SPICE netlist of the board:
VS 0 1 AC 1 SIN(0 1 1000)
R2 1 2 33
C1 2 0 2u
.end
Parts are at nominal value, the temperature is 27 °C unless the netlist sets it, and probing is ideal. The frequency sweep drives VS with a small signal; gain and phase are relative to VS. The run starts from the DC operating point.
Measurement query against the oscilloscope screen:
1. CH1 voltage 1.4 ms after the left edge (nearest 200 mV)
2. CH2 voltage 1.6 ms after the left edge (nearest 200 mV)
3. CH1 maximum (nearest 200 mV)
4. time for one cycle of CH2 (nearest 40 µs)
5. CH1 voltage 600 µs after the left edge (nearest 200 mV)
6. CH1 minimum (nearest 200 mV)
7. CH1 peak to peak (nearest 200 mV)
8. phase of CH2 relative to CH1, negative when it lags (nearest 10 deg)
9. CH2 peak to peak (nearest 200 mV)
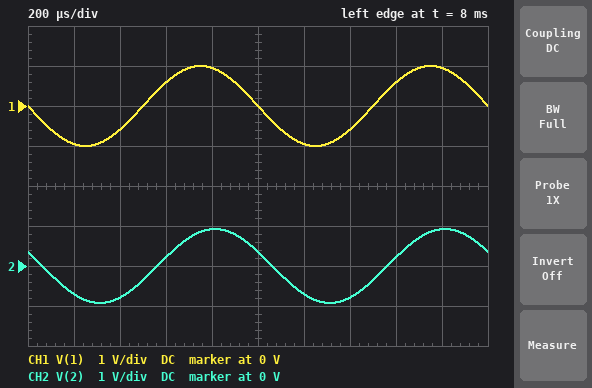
-600 mV
200 mV
1.0 V
1.00 ms
600 mV
-1.0 V
2.0 V
-20 deg
1.8 V
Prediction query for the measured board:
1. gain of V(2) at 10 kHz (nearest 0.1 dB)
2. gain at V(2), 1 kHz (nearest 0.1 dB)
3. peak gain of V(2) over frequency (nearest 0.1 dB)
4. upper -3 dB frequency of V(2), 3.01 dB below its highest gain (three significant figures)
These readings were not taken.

-12.6 dB
-0.7 dB
0 dB
2.41 kHz
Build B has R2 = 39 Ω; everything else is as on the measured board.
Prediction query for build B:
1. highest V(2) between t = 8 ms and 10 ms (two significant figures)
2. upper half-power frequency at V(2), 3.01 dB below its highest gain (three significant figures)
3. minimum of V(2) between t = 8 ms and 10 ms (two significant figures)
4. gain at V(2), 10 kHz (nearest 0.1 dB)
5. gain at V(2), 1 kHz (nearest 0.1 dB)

900 mV
2.04 kHz
-900 mV
-14.0 dB
-0.9 dB
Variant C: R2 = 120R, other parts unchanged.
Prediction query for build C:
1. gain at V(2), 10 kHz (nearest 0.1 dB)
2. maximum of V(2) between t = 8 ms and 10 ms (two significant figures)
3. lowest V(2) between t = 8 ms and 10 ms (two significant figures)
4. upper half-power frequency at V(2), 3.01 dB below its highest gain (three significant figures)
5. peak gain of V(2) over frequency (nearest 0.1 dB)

-23.6 dB
550 mV
-550 mV
663 Hz
0 dB
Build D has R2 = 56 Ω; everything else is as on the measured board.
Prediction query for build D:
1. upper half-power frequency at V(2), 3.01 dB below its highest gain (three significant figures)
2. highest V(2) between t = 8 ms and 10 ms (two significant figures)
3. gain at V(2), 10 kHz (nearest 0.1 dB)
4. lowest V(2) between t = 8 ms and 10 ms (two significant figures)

1.42 kHz
820 mV
-17.0 dB
-820 mV
